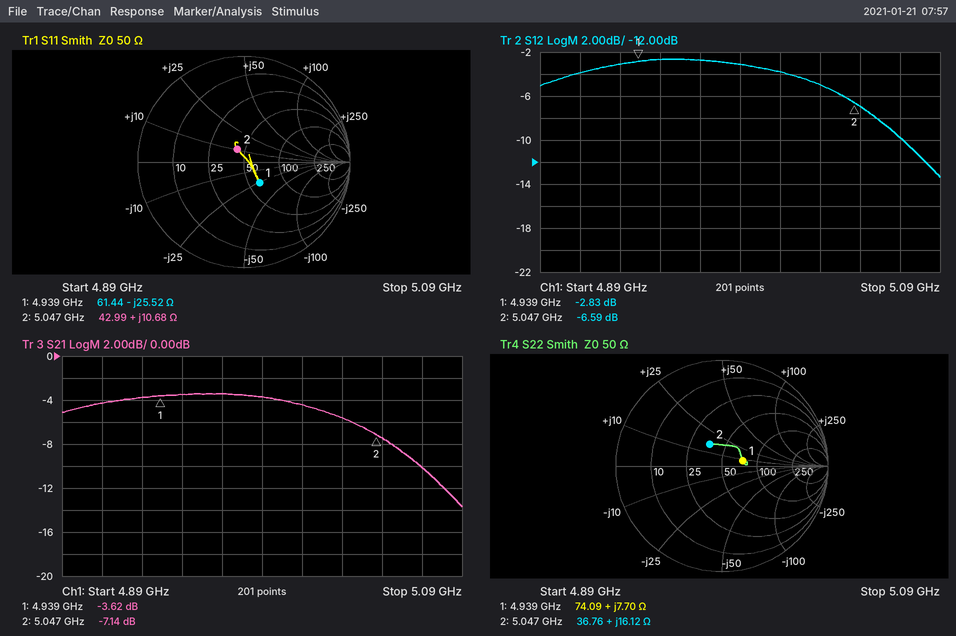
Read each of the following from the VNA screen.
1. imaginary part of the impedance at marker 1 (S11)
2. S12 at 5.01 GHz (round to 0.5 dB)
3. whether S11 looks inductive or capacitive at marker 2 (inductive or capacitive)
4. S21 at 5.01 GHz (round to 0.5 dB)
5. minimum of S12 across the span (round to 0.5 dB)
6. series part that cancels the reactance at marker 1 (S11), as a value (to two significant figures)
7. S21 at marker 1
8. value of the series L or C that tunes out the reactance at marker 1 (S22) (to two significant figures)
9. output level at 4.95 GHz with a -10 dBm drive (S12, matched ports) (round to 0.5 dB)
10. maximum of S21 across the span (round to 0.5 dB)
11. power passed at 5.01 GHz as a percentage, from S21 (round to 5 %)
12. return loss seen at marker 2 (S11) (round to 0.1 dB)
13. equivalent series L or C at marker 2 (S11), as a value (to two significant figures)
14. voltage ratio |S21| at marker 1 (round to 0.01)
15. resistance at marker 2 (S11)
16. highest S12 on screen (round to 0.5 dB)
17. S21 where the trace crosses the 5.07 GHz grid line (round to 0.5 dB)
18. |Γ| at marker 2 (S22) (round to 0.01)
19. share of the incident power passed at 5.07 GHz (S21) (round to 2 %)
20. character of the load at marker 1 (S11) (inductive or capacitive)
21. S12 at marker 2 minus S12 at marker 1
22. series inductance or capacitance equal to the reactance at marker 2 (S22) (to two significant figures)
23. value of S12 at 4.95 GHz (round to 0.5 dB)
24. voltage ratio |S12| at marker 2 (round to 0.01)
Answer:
-25.52 Ω
-4.0 dB
inductive
-4.5 dB
-13.5 dB
820 pH
-3.62 dB
4.2 pF
-12.5 dBm
-3.5 dB
35 %
17.3 dB
340 pH
0.66
42.99 Ω
-2.5 dB
-10.0 dB
0.24
10 %
capacitive
-3.76 dB
510 pH
-2.5 dB
0.47
